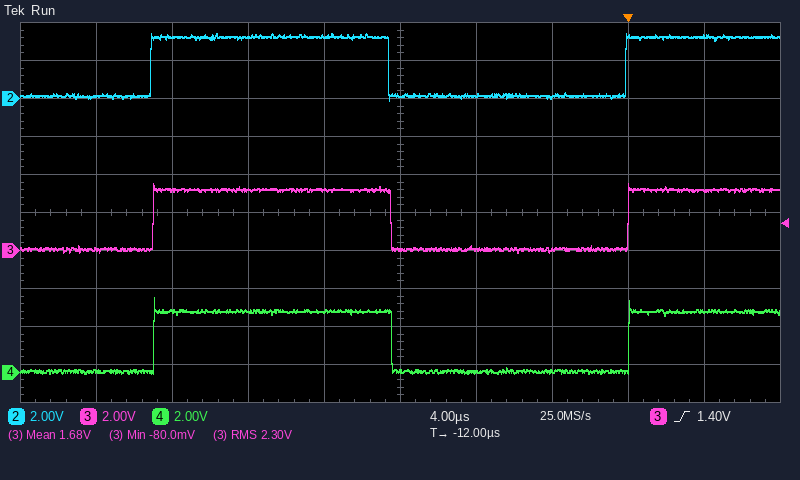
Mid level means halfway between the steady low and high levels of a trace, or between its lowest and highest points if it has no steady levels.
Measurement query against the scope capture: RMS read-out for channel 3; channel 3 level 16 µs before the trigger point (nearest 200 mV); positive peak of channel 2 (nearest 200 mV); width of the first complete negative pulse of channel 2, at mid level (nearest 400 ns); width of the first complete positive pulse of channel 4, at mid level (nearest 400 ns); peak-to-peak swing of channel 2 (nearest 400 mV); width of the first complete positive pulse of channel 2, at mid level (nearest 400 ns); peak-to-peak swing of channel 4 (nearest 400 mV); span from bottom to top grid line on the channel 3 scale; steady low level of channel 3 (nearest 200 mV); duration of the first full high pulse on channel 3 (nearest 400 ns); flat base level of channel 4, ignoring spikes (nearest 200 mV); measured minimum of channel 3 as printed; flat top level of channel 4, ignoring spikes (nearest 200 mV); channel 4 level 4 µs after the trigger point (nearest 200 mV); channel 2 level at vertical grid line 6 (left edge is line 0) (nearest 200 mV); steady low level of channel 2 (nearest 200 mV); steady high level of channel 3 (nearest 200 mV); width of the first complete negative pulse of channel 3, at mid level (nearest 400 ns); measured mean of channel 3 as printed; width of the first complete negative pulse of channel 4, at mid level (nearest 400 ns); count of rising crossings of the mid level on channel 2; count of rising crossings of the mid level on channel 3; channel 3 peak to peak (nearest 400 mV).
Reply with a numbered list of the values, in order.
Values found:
1. 2.30 V
2. 3.2 V
3. 3.4 V
4. 12.4 µs
5. 12.4 µs
6. 3.6 V
7. 12.4 µs
8. 4.0 V
9. 20 V
10. 0.0 V
11. 12.4 µs
12. 0.0 V
13. -80.0 mV
14. 3.2 V
15. 3.2 V
16. 200 mV
17. 200 mV
18. 3.2 V
19. 12.4 µs
20. 1.68 V
21. 12.4 µs
22. 2
23. 2
24. 3.6 V
